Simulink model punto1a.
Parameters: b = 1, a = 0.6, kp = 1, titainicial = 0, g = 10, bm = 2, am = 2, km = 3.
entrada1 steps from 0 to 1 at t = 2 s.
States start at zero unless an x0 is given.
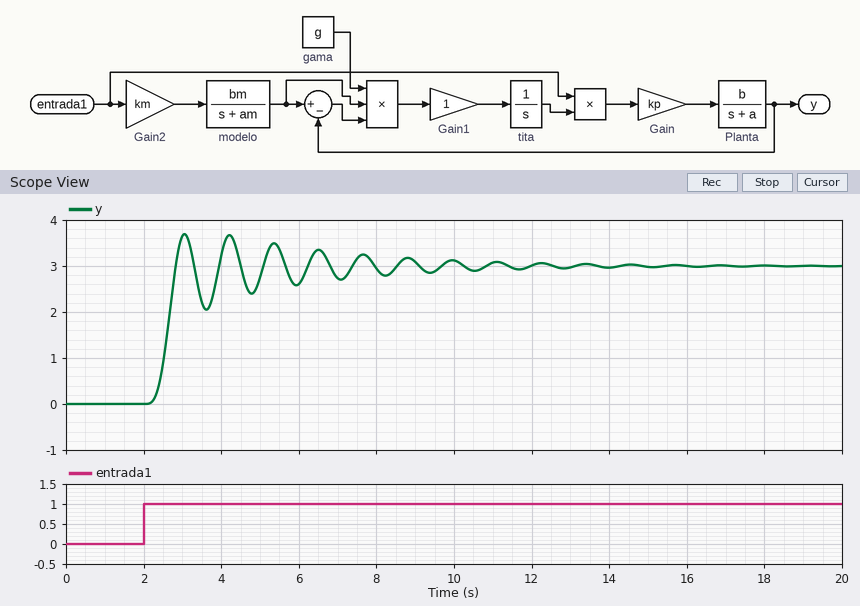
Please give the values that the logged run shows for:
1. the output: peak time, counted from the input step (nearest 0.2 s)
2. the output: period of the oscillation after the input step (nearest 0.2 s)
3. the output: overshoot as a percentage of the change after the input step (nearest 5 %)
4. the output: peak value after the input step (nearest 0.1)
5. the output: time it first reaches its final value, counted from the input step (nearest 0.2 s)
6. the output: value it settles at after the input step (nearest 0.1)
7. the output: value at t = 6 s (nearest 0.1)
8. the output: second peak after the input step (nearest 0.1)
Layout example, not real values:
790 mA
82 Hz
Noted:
1.0 s
1.2 s
25 %
3.7
0.8 s
3.0
2.6
3.7
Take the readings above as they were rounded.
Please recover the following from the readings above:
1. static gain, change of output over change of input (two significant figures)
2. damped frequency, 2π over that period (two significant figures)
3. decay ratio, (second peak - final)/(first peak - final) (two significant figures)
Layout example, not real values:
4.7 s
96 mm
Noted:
3.0
5.2 rad/s
1.0
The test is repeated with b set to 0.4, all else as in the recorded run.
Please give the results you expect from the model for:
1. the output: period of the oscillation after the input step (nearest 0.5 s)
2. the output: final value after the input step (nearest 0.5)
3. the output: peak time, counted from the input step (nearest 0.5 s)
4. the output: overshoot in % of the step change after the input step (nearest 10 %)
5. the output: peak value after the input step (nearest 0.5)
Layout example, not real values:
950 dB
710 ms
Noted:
2.0 s
3.0
1.5 s
40 %
4.0
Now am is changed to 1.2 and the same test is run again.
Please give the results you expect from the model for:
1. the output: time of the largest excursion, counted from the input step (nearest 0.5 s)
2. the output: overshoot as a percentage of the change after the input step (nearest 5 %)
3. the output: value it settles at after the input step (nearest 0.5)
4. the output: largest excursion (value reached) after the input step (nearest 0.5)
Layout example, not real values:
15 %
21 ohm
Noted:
3.0 s
10 %
5.0
5.5
